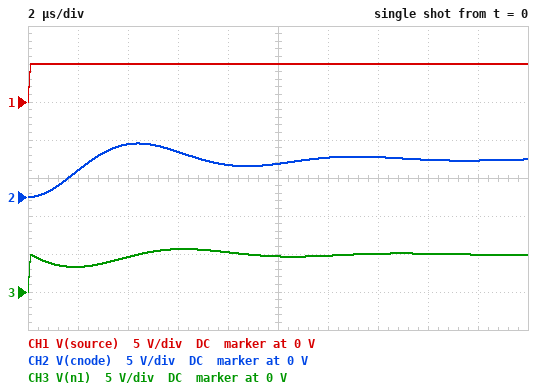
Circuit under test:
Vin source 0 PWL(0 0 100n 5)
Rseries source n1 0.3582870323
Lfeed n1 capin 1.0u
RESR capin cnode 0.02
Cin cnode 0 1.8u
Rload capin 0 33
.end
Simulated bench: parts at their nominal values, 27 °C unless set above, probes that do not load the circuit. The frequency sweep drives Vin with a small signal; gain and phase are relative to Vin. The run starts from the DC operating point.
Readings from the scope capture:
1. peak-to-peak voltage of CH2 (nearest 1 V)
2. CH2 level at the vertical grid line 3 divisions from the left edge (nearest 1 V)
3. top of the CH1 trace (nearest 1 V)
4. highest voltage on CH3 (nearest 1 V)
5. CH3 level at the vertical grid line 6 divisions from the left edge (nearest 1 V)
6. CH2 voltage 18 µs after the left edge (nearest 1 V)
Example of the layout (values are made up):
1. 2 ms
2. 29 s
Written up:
1. 7 V
2. 6 V
3. 5 V
4. 6 V
5. 5 V
6. 5 V
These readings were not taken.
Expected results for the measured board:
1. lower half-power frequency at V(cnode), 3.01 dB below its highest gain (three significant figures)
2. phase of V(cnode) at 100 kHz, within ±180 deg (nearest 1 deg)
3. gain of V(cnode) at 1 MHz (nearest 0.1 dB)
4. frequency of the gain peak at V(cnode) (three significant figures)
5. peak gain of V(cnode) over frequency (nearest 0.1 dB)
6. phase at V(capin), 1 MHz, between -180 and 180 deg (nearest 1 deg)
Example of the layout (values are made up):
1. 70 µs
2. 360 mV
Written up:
1. 70.8 kHz
2. -56 deg
3. -36.9 dB
4. 111 kHz
5. 5.8 dB
6. -164 deg
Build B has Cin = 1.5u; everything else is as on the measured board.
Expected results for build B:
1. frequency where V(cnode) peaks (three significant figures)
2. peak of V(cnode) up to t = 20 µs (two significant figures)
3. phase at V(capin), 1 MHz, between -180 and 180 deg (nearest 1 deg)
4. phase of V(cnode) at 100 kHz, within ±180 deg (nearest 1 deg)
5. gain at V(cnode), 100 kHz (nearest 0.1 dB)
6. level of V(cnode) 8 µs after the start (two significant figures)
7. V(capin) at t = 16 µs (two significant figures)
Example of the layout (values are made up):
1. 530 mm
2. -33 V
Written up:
1. 123 kHz
2. 7.2 V
3. -166 deg
4. -42 deg
5. 5.0 dB
6. 3.9 V
7. 4.7 V
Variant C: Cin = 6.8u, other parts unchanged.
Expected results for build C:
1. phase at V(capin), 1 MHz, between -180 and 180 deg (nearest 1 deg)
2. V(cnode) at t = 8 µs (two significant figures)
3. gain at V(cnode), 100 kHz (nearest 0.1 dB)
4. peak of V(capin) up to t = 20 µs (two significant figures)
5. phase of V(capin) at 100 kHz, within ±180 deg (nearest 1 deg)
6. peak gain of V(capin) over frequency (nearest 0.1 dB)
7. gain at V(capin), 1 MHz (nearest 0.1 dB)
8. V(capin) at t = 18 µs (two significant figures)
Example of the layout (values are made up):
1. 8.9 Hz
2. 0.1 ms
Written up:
1. -136 deg
2. 5.6 V
3. -7.4 dB
4. 5.8 V
5. -131 deg
6. 1.2 dB
7. -46.2 dB
8. 4.8 V
